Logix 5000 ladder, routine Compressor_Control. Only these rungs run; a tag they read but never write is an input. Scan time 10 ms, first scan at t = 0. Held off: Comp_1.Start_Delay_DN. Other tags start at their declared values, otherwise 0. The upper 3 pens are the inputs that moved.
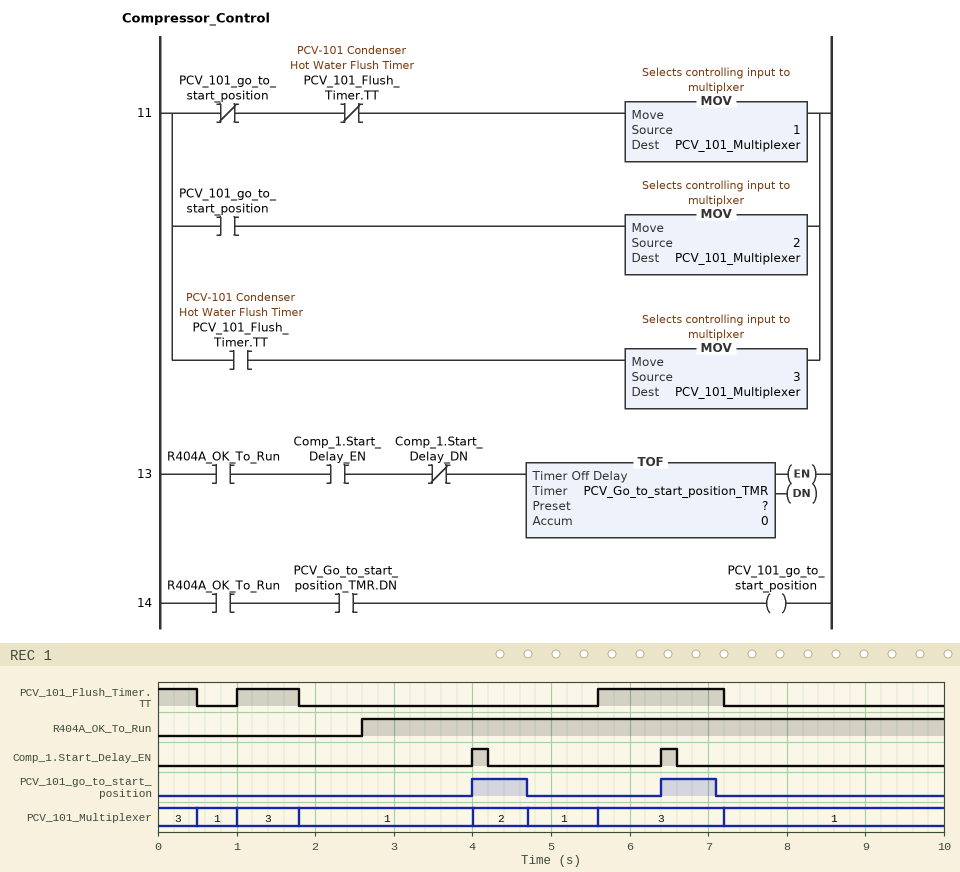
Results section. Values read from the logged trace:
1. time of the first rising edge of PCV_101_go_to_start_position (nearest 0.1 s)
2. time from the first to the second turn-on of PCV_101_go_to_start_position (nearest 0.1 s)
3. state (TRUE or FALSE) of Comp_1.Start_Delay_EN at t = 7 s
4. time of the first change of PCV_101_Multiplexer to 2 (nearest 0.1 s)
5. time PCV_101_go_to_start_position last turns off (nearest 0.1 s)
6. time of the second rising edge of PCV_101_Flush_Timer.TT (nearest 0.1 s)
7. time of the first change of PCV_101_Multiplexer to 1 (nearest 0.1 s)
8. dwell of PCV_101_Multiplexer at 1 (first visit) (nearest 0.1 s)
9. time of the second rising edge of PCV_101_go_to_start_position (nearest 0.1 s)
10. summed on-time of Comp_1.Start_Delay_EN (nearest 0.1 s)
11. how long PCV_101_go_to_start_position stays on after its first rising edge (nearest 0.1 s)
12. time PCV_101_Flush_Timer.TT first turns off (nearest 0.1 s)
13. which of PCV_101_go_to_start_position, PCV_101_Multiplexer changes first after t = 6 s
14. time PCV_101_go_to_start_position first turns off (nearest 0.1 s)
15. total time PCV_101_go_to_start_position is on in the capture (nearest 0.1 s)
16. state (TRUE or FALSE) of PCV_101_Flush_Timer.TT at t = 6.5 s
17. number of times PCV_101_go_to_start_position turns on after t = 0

4.0 s
2.4 s
FALSE
4.0 s
7.1 s
5.6 s
0.5 s
0.5 s
6.4 s
0.4 s
0.7 s
0.5 s
PCV_101_go_to_start_position
4.7 s
1.4 s
TRUE
2
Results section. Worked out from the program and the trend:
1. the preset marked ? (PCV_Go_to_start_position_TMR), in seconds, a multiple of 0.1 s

0.5 s
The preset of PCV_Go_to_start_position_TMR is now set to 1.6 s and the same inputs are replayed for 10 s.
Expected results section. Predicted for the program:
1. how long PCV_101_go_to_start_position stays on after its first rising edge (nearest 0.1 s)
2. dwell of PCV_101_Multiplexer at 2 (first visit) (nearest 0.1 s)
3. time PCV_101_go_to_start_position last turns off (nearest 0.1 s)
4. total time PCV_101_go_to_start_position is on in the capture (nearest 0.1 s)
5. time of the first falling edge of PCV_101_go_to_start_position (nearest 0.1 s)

1.8 s
1.6 s
8.2 s
3.6 s
5.8 s
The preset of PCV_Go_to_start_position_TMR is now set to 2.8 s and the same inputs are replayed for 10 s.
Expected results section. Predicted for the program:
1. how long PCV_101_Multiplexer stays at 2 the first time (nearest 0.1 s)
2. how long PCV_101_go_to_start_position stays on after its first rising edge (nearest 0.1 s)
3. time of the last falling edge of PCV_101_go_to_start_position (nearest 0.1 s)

1.6 s
5.4 s
9.4 s
